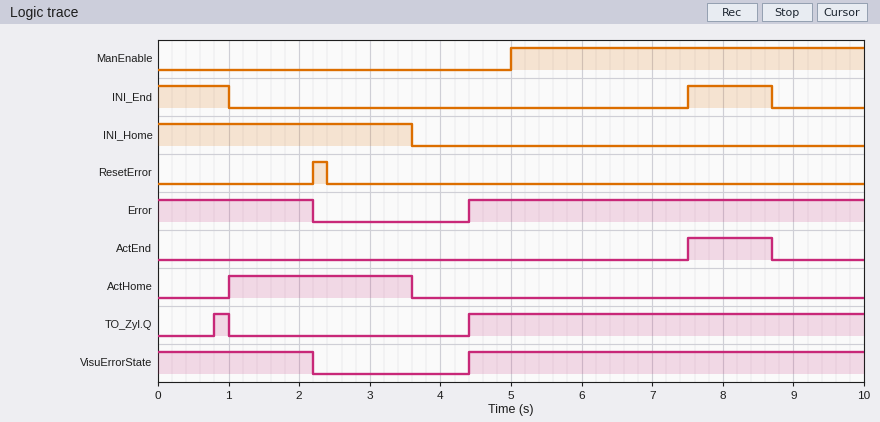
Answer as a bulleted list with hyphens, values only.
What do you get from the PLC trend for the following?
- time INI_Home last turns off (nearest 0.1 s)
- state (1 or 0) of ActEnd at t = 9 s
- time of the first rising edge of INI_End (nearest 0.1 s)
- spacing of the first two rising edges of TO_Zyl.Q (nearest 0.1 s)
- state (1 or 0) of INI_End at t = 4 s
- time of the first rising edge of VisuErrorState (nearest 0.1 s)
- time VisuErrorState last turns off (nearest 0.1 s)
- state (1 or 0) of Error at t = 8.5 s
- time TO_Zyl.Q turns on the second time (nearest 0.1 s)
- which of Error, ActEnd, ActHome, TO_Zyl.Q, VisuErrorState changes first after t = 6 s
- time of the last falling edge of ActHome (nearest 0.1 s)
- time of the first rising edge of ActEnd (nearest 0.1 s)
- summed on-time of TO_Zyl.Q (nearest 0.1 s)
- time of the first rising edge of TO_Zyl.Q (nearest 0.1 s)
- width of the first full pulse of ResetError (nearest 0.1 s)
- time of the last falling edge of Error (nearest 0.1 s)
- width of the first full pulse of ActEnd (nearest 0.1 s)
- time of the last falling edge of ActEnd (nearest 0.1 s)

- 3.6 s
- 0
- 7.5 s
- 3.6 s
- 0
- 4.4 s
- 2.2 s
- 1
- 4.4 s
- ActEnd
- 3.6 s
- 7.5 s
- 5.8 s
- 0.8 s
- 0.2 s
- 2.2 s
- 1.2 s
- 8.7 s
